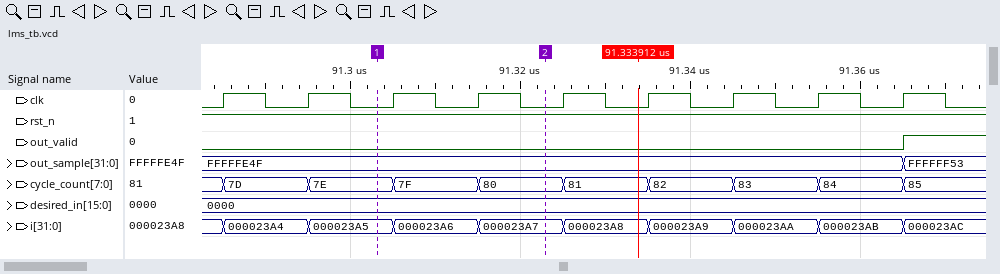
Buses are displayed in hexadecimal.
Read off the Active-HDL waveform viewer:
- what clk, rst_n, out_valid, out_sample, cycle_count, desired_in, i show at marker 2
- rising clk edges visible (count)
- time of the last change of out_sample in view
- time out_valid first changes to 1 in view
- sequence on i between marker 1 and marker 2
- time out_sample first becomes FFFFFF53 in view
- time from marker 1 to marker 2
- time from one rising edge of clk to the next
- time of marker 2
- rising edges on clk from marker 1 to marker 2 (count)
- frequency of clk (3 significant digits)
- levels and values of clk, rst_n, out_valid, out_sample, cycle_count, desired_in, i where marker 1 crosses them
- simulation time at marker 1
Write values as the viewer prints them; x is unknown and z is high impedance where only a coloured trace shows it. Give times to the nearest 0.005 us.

clk=0, rst_n=1, out_valid=0, out_sample=FFFFFE4F, cycle_count=80, desired_in=0000, i=000023A7
9
91.365 us
91.365 us
000023A5, 000023A6, 000023A7
91.365 us
0.02 us
0.01 us
91.325 us
2
100 MHz
clk=0, rst_n=1, out_valid=0, out_sample=FFFFFE4F, cycle_count=7E, desired_in=0000, i=000023A5
91.305 us
